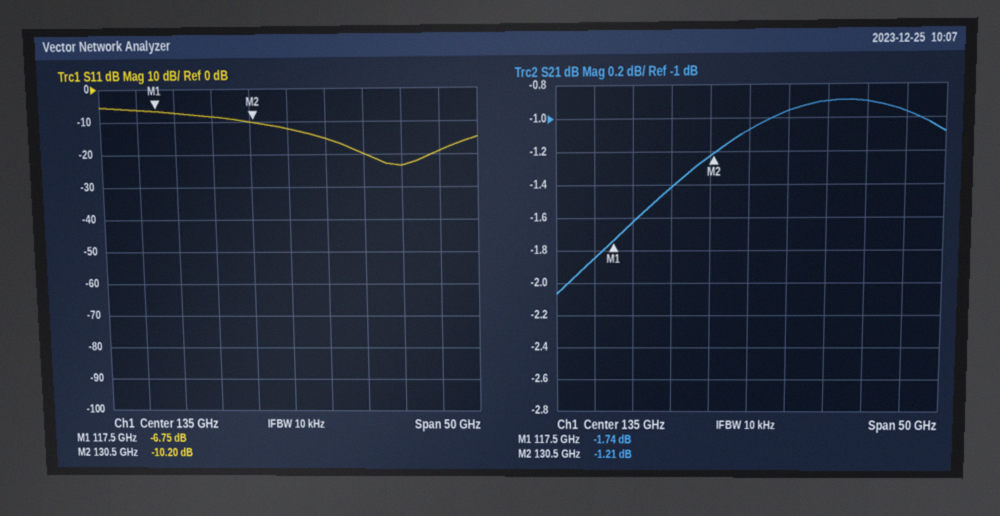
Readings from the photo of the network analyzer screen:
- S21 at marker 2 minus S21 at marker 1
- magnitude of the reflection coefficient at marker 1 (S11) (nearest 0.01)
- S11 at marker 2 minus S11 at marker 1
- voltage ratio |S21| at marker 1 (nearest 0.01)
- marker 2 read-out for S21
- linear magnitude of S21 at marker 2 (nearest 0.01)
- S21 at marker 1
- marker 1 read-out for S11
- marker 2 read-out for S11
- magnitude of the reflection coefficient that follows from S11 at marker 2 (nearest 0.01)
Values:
0.53 dB
0.46
-3.45 dB
0.82
-1.21 dB
0.87
-1.74 dB
-6.75 dB
-10.20 dB
0.31
